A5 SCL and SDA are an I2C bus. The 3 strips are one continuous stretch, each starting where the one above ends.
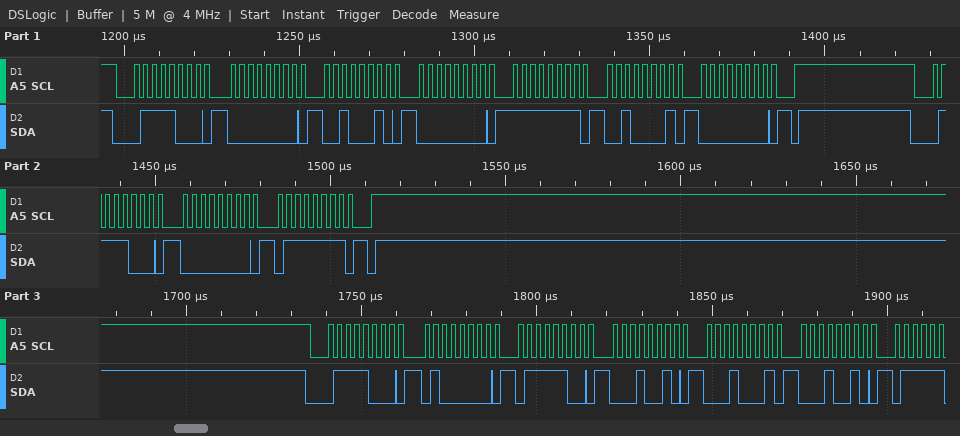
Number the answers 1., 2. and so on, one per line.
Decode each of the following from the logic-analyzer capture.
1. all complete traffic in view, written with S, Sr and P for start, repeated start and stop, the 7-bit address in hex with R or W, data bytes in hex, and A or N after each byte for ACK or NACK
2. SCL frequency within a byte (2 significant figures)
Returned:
1. S 3CW A 00 A 22 A 00 A FF A 21 A 00 A P S 3CW A 00 A 7F A P S 3CW A 40 A 7C A 12 A 11 A 12 A
2. 400 kHz
